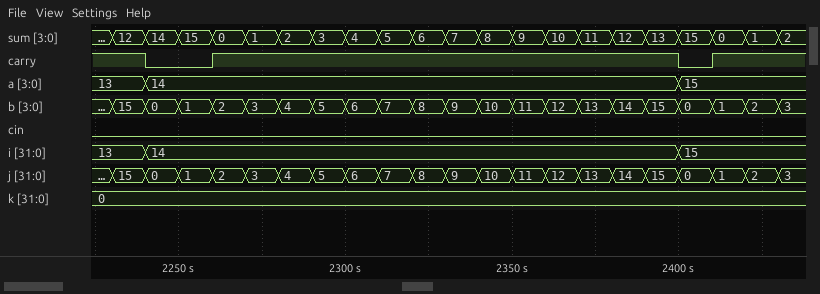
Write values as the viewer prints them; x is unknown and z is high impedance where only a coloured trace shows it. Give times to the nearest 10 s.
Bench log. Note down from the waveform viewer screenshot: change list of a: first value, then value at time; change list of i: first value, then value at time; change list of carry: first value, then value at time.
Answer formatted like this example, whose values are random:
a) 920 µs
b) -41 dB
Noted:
a) 13, 14 at 2240 s, 15 at 2400 s
b) 13, 14 at 2240 s, 15 at 2400 s
c) 1, 0 at 2240 s, 1 at 2260 s, 0 at 2400 s, 1 at 2410 s
